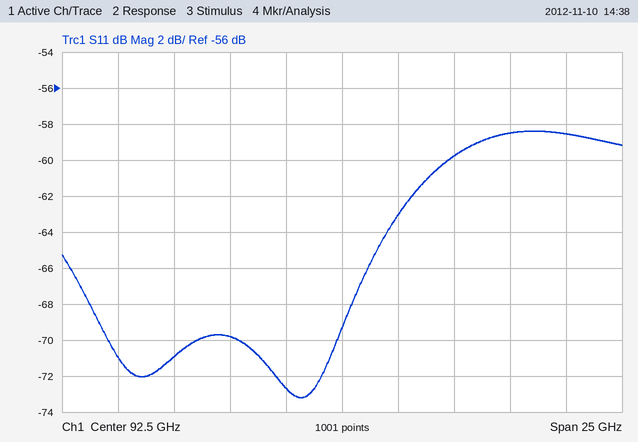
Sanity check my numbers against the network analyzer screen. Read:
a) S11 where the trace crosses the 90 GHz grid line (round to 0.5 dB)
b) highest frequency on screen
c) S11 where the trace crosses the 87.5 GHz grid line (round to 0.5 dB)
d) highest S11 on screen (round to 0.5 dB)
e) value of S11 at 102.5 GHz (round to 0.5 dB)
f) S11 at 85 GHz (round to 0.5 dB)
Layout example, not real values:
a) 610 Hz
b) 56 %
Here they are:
a) -72.5 dB
b) 105 GHz
c) -70.0 dB
d) -58.5 dB
e) -58.5 dB
f) -71.0 dB
